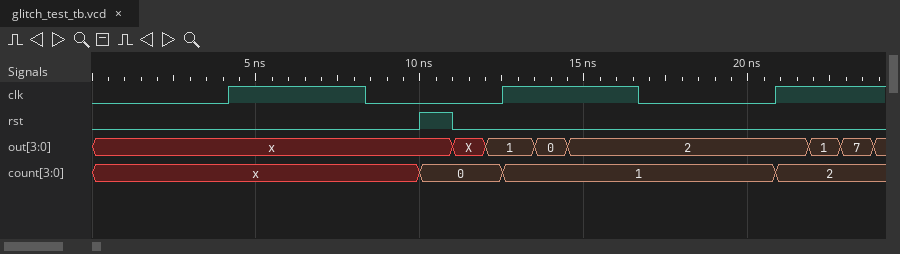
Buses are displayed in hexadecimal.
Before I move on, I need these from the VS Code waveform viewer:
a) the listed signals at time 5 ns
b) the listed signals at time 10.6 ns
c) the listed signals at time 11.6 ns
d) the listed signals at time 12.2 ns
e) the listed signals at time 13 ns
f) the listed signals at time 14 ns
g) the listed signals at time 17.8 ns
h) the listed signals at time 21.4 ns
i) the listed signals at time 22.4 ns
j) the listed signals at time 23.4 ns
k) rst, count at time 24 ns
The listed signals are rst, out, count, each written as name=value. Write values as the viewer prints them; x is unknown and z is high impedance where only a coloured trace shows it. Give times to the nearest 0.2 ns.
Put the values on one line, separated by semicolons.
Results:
rst=0, out=x, count=x; rst=1, out=x, count=0; rst=0, out=X, count=0; rst=0, out=1, count=0; rst=0, out=1, count=1; rst=0, out=0, count=1; rst=0, out=2, count=1; rst=0, out=2, count=2; rst=0, out=1, count=2; rst=0, out=7, count=2; rst=0, count=2
